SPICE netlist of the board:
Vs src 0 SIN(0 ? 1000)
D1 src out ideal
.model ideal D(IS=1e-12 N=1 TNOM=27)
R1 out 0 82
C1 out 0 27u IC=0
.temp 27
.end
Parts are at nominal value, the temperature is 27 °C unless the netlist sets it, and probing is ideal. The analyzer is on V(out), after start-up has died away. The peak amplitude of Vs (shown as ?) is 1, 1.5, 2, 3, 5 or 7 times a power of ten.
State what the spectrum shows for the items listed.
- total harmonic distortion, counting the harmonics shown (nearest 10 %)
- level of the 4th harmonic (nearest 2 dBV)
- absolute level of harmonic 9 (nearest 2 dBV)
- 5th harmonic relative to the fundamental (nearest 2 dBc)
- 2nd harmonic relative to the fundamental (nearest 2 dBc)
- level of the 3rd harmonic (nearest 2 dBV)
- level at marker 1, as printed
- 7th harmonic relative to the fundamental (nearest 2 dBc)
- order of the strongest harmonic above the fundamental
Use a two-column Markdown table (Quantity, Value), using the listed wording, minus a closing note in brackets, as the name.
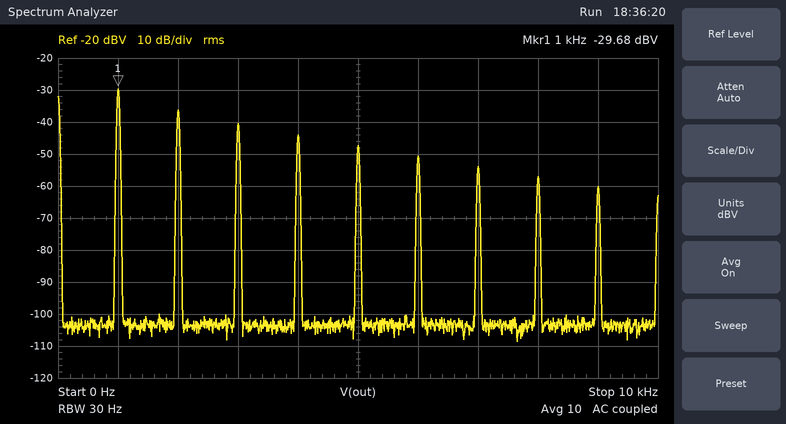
| Quantity | Value |
|---|---|
| total harmonic distortion, counting the harmonics shown | 60 % |
| level of the 4th harmonic | -44 dBV |
| absolute level of harmonic 9 | -60 dBV |
| 5th harmonic relative to the fundamental | -18 dBc |
| 2nd harmonic relative to the fundamental | -6 dBc |
| level of the 3rd harmonic | -40 dBV |
| level at marker 1, as printed | -29.68 dBV |
| 7th harmonic relative to the fundamental | -24 dBc |
| order of the strongest harmonic above the fundamental | 2 |
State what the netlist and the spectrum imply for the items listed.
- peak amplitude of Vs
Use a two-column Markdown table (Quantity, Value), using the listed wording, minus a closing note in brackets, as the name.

| Quantity | Value |
|---|---|
| peak amplitude of Vs | 1 V |
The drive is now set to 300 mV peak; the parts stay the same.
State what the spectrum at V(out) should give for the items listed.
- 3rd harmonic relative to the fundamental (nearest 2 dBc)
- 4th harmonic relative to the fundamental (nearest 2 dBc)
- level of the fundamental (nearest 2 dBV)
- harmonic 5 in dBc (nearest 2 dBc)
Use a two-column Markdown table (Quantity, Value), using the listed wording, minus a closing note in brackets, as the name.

| Quantity | Value |
|---|---|
| 3rd harmonic relative to the fundamental | -12 dBc |
| 4th harmonic relative to the fundamental | -18 dBc |
| level of the fundamental | -140 dBV |
| harmonic 5 in dBc | -24 dBc |
